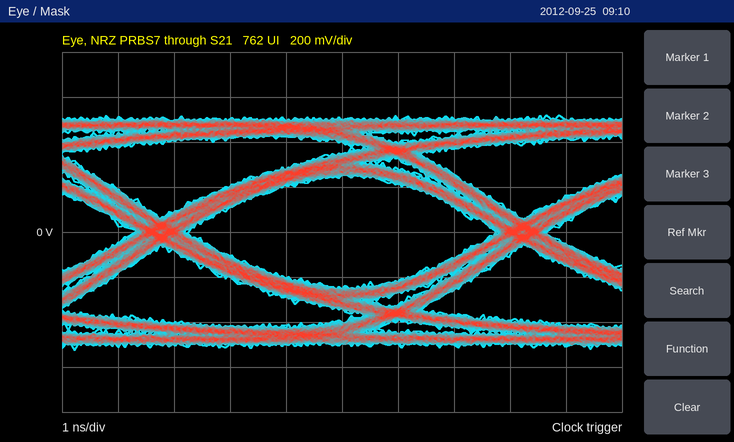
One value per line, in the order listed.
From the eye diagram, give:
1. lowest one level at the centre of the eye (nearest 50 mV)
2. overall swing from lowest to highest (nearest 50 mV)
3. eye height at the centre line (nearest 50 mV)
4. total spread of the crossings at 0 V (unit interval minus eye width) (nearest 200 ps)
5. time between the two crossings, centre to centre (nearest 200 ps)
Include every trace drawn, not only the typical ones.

250 mV
1.05 V
500 mV
1.0 ns
6.4 ns
